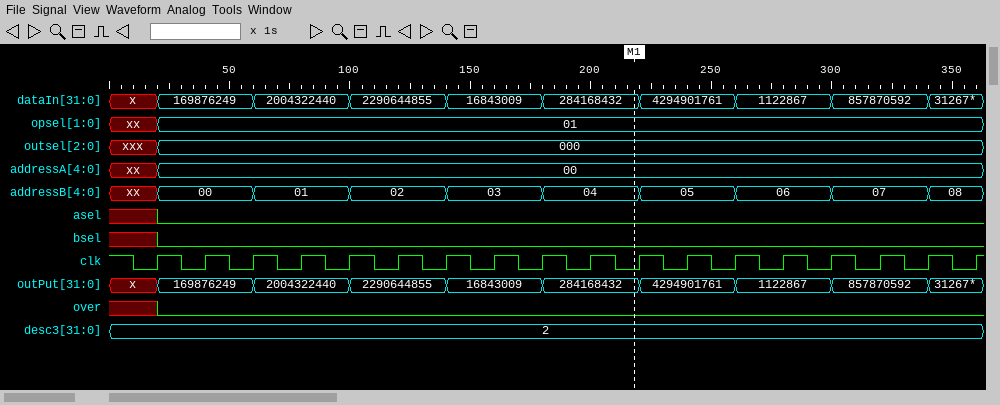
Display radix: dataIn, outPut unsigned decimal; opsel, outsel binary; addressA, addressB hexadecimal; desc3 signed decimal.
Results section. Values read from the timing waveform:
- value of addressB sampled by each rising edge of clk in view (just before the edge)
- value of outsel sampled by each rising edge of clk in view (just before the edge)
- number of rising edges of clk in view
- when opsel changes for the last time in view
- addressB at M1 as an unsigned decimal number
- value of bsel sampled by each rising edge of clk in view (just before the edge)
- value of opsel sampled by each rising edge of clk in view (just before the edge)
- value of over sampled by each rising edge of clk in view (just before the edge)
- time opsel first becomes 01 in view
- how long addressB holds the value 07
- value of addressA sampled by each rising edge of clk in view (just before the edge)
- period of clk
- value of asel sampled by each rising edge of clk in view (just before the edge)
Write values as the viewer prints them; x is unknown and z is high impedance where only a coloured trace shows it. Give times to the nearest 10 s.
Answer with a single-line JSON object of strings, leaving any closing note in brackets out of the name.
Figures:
{"value of addressB sampled by each rising edge of clk in view": "xx, 00, 00, 01, 01, 02, 02, 03, 03, 04, 04, 05, 05, 06, 06, 07, 07, 08", "value of outsel sampled by each rising edge of clk in view": "xxx, 000, 000, 000, 000, 000, 000, 000, 000, 000, 000, 000, 000, 000, 000, 000, 000, 000", "number of rising edges of clk in view": "18", "when opsel changes for the last time in view": "20 s", "addressB at M1 as an unsigned decimal number": "4", "value of bsel sampled by each rising edge of clk in view": "x 0 0 0 0 0 0 0 0 0 0 0 0 0 0 0 0 0", "value of opsel sampled by each rising edge of clk in view": "xx, 01, 01, 01, 01, 01, 01, 01, 01, 01, 01, 01, 01, 01, 01, 01, 01, 01", "value of over sampled by each rising edge of clk in view": "x 0 0 0 0 0 0 0 0 0 0 0 0 0 0 0 0 0", "time opsel first becomes 01 in view": "20 s", "how long addressB holds the value 07": "40 s", "value of addressA sampled by each rising edge of clk in view": "xx, 00, 00, 00, 00, 00, 00, 00, 00, 00, 00, 00, 00, 00, 00, 00, 00, 00", "period of clk": "20 s", "value of asel sampled by each rising edge of clk in view": "x 0 0 0 0 0 0 0 0 0 0 0 0 0 0 0 0 0"}
